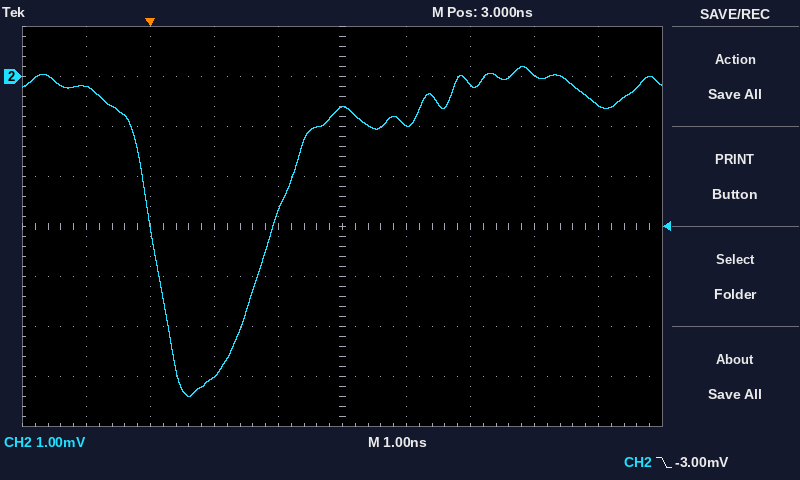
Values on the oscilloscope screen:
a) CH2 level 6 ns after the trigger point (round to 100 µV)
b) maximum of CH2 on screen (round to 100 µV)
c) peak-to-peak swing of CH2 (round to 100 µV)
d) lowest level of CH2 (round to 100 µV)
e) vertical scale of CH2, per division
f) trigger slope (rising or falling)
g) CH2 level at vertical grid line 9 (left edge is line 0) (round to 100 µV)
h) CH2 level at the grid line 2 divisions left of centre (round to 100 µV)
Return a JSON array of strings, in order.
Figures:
["0.0 mV", "200 µV", "6.6 mV", "-6.4 mV", "1 mV", "falling", "-600 µV", "-6.0 mV"]
